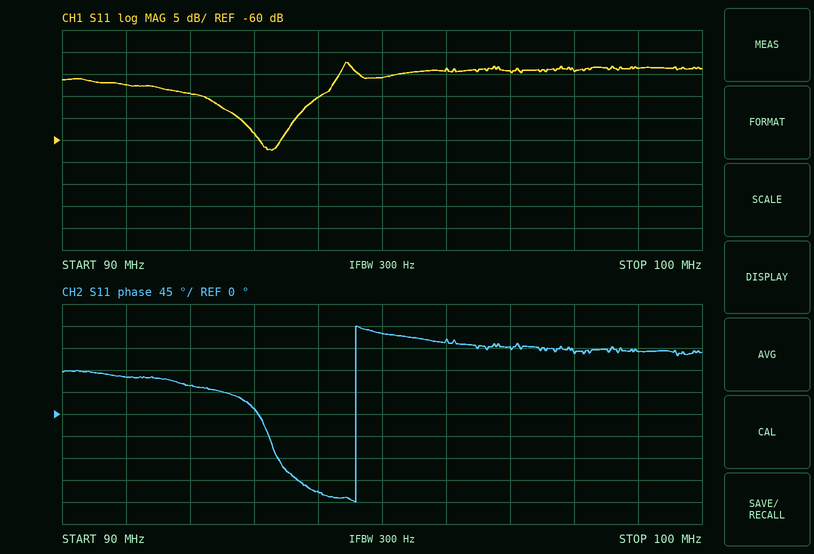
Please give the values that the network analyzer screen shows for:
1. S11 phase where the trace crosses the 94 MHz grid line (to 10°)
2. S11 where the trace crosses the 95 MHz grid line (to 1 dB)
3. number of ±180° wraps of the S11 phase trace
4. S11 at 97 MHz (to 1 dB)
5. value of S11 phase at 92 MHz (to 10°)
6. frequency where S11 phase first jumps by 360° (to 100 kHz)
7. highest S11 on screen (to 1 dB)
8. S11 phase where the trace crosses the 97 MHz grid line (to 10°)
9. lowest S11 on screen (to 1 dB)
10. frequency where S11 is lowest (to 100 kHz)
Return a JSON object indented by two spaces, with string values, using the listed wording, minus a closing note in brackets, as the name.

{
  "S11 phase where the trace crosses the 94 MHz grid line": "-160°",
  "S11 where the trace crosses the 95 MHz grid line": "-46 dB",
  "number of ±180° wraps of the S11 phase trace": "1",
  "S11 at 97 MHz": "-44 dB",
  "value of S11 phase at 92 MHz": "60°",
  "frequency where S11 phase first jumps by 360°": "94.6 MHz",
  "highest S11 on screen": "-42 dB",
  "S11 phase where the trace crosses the 97 MHz grid line": "140°",
  "lowest S11 on screen": "-62 dB",
  "frequency where S11 is lowest": "93.3 MHz"
}
